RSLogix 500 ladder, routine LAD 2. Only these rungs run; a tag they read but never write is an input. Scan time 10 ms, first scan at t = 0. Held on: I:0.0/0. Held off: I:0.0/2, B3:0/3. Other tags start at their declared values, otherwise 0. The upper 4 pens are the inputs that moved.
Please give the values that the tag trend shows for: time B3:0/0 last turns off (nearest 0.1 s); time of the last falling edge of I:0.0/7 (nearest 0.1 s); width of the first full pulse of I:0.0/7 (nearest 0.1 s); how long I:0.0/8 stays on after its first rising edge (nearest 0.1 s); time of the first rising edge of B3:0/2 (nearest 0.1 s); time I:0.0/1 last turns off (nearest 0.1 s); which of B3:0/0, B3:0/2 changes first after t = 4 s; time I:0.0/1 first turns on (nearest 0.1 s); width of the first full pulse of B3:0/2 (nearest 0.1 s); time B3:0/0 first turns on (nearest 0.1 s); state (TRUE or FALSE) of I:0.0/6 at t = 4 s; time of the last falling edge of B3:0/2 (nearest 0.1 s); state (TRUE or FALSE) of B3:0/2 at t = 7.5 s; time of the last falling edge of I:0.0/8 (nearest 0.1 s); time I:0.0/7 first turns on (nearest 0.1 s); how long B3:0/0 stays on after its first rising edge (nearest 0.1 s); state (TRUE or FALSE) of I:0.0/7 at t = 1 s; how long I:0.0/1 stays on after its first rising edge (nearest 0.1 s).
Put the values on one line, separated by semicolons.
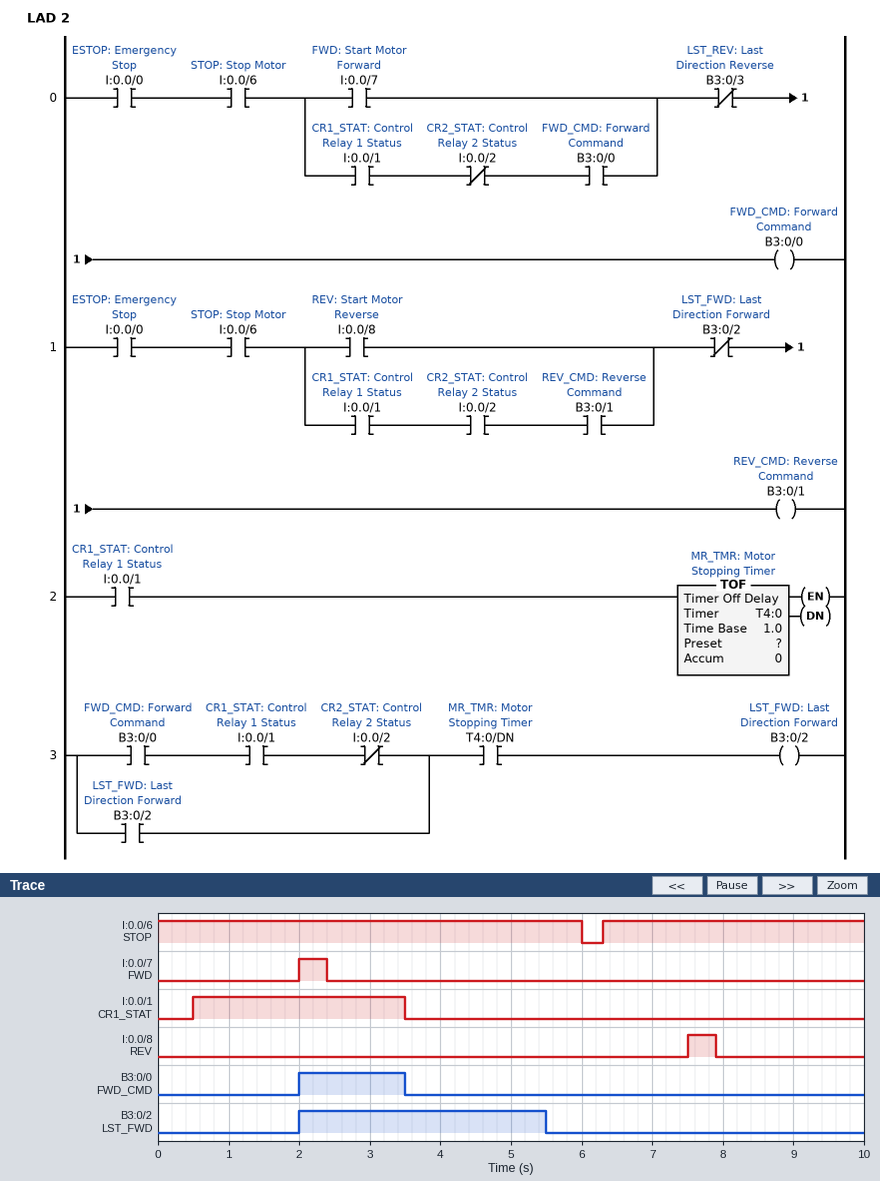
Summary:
3.5 s; 2.4 s; 0.4 s; 0.4 s; 2.0 s; 3.5 s; B3:0/2; 0.5 s; 3.5 s; 2.0 s; TRUE; 5.5 s; FALSE; 7.9 s; 2.0 s; 1.5 s; FALSE; 3.0 s
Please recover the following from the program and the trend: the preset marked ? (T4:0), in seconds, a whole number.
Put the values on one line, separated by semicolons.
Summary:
2 s
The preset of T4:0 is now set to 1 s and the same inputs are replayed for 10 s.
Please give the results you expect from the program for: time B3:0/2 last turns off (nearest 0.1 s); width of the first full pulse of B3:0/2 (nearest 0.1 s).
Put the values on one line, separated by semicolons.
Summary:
4.5 s; 2.5 s
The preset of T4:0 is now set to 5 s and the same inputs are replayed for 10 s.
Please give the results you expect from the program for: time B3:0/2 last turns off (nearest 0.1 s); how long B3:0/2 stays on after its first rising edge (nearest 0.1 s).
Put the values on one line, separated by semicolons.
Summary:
8.5 s; 6.5 s
